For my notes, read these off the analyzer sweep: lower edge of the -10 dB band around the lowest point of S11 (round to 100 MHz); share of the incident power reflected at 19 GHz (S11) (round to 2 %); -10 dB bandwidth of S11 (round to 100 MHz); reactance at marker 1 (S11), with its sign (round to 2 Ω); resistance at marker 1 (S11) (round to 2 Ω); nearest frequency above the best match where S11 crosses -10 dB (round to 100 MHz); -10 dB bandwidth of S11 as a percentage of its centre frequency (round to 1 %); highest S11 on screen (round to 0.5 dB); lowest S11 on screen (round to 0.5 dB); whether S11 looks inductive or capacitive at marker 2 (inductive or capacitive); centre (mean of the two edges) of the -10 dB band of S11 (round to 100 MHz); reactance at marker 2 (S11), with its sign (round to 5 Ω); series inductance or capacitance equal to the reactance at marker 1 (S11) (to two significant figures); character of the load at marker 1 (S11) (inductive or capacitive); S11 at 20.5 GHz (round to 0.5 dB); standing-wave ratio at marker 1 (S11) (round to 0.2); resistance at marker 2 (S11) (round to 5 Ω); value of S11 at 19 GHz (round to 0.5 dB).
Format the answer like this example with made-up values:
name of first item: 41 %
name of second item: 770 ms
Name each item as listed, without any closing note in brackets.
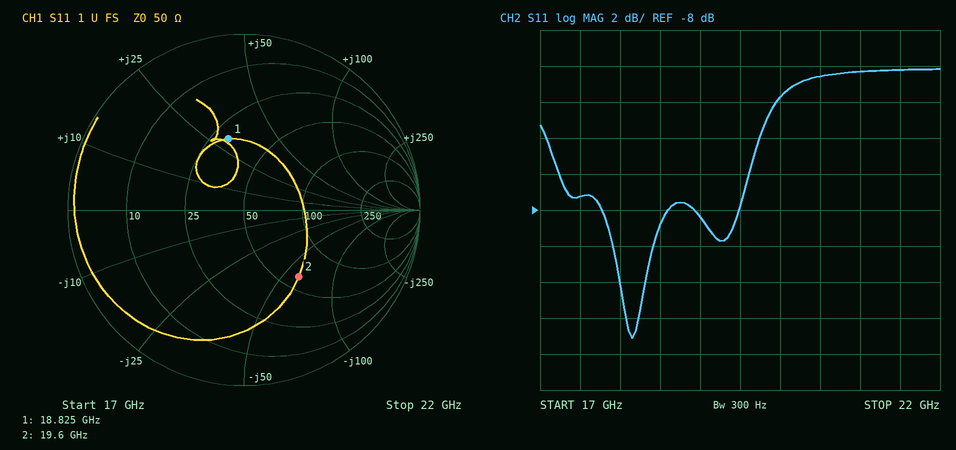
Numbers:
lower edge of the -10 dB band around the lowest point of S11: 17.9 GHz
share of the incident power reflected at 19 GHz (S11): 14 %
-10 dB bandwidth of S11: 500 MHz
reactance at marker 1 (S11), with its sign: +30 Ω
resistance at marker 1 (S11): 30 Ω
nearest frequency above the best match where S11 crosses -10 dB: 18.4 GHz
-10 dB bandwidth of S11 as a percentage of its centre frequency: 3 %
highest S11 on screen: 0.0 dB
lowest S11 on screen: -15.0 dB
whether S11 looks inductive or capacitive at marker 2: capacitive
centre (mean of the two edges) of the -10 dB band of S11: 18.2 GHz
reactance at marker 2 (S11), with its sign: -60 Ω
series inductance or capacitance equal to the reactance at marker 1 (S11): 250 pH
character of the load at marker 1 (S11): inductive
S11 at 20.5 GHz: -0.5 dB
standing-wave ratio at marker 1 (S11): 2.4
resistance at marker 2 (S11): 60 Ω
value of S11 at 19 GHz: -8.5 dB
